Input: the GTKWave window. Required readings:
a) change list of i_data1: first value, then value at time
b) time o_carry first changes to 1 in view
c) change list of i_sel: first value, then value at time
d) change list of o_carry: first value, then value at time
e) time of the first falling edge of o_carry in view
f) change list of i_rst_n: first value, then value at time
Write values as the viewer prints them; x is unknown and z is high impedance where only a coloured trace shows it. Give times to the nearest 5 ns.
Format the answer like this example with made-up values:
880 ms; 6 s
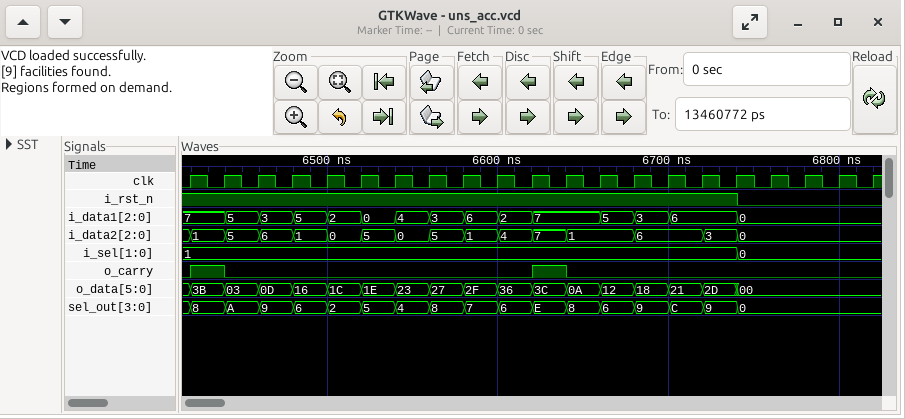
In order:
7, 5 at 6440 ns, 3 at 6460 ns, 5 at 6480 ns, 2 at 6500 ns, 0 at 6520 ns, 4 at 6540 ns, 3 at 6560 ns, 6 at 6580 ns, 2 at 6600 ns, 7 at 6620 ns, 5 at 6660 ns, 3 at 6680 ns, 6 at 6700 ns, 0 at 6740 ns; 6420 ns; 1, 0 at 6740 ns; 0, 1 at 6420 ns, 0 at 6440 ns, 1 at 6620 ns, 0 at 6640 ns; 6440 ns; 1, 0 at 6740 ns
